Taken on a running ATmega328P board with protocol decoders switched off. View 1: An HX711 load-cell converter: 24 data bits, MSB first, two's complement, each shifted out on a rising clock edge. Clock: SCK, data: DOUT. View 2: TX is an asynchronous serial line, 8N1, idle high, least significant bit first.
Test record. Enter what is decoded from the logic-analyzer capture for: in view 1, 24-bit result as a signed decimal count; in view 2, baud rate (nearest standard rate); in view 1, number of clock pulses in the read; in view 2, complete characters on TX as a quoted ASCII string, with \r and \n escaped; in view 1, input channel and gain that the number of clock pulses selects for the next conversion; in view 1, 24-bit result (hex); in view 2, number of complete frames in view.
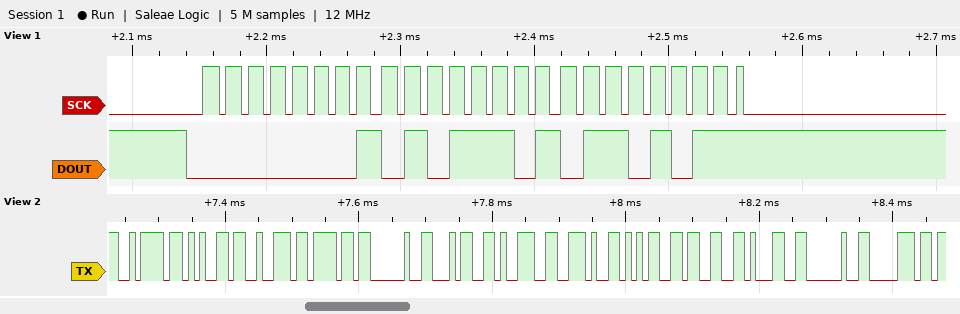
89451
115200 baud
25
"zero 49.531 p"
channel A, gain 128
0x015D6B
13
